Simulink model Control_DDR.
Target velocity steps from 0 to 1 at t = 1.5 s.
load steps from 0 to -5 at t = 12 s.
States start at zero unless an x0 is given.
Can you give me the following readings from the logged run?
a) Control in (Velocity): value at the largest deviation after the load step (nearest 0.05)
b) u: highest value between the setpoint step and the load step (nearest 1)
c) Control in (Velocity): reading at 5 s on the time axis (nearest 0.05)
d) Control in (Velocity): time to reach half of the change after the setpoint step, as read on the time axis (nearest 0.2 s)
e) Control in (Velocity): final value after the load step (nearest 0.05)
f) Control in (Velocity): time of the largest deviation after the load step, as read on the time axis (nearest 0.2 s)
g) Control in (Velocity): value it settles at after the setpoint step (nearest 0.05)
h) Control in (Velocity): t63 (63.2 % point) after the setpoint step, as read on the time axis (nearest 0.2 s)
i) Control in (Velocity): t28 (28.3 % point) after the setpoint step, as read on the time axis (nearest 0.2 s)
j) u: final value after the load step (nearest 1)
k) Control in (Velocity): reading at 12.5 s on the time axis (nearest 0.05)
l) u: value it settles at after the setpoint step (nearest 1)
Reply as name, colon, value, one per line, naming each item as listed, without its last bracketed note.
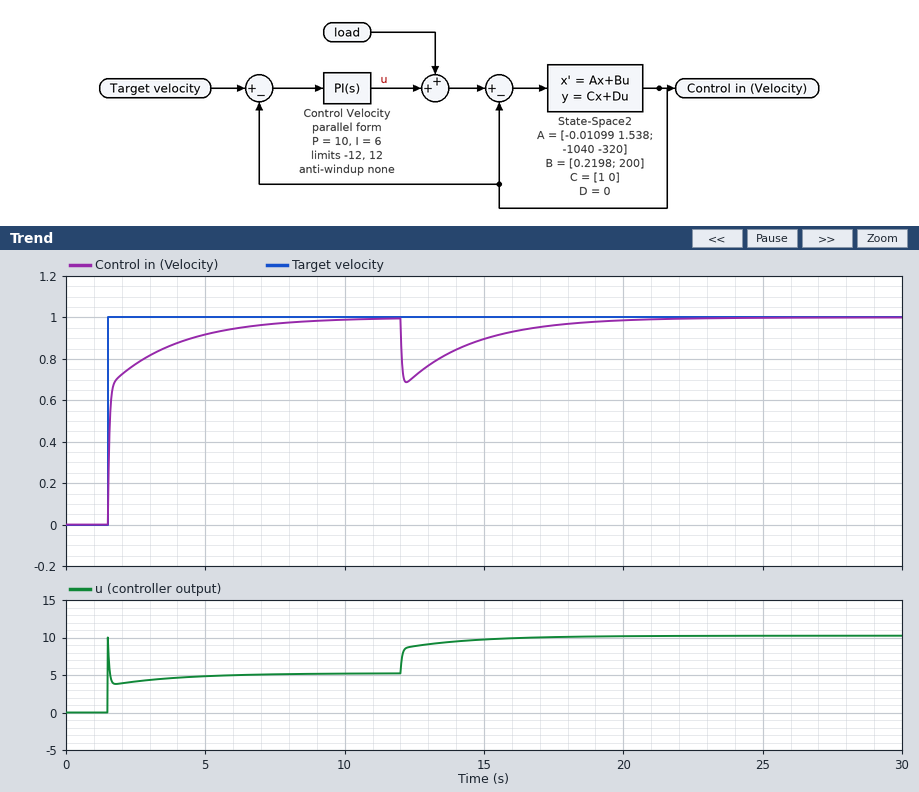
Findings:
Control in (Velocity): value at the largest deviation after the load step: 0.70
u: highest value between the setpoint step and the load step: 10
Control in (Velocity): reading at 5 s on the time axis: 0.90
Control in (Velocity): time to reach half of the change after the setpoint step, as read on the time axis: 1.6 s
Control in (Velocity): final value after the load step: 1.00
Control in (Velocity): time of the largest deviation after the load step, as read on the time axis: 12.2 s
Control in (Velocity): value it settles at after the setpoint step: 1.00
Control in (Velocity): t63 (63.2 % point) after the setpoint step, as read on the time axis: 1.6 s
Control in (Velocity): t28 (28.3 % point) after the setpoint step, as read on the time axis: 1.6 s
u: final value after the load step: 10
Control in (Velocity): reading at 12.5 s on the time axis: 0.70
u: value it settles at after the setpoint step: 5
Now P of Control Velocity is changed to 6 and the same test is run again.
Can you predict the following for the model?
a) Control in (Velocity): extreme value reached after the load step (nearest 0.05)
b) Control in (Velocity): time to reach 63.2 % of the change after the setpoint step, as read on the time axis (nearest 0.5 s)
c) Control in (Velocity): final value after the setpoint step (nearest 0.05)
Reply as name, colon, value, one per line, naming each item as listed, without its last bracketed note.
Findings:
Control in (Velocity): extreme value reached after the load step: 0.60
Control in (Velocity): time to reach 63.2 % of the change after the setpoint step, as read on the time axis: 2.0 s
Control in (Velocity): final value after the setpoint step: 1.00
